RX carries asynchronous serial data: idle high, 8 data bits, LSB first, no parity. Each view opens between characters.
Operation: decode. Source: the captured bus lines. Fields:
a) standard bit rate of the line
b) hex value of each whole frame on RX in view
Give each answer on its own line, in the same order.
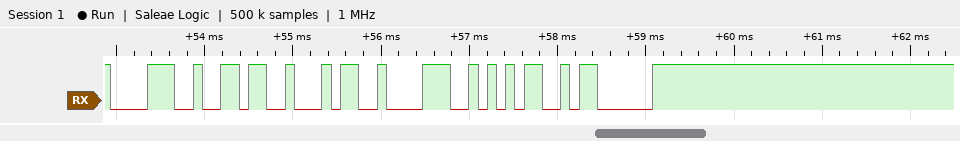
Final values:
9600 baud
38, 36, 34, 38, 35, 03
